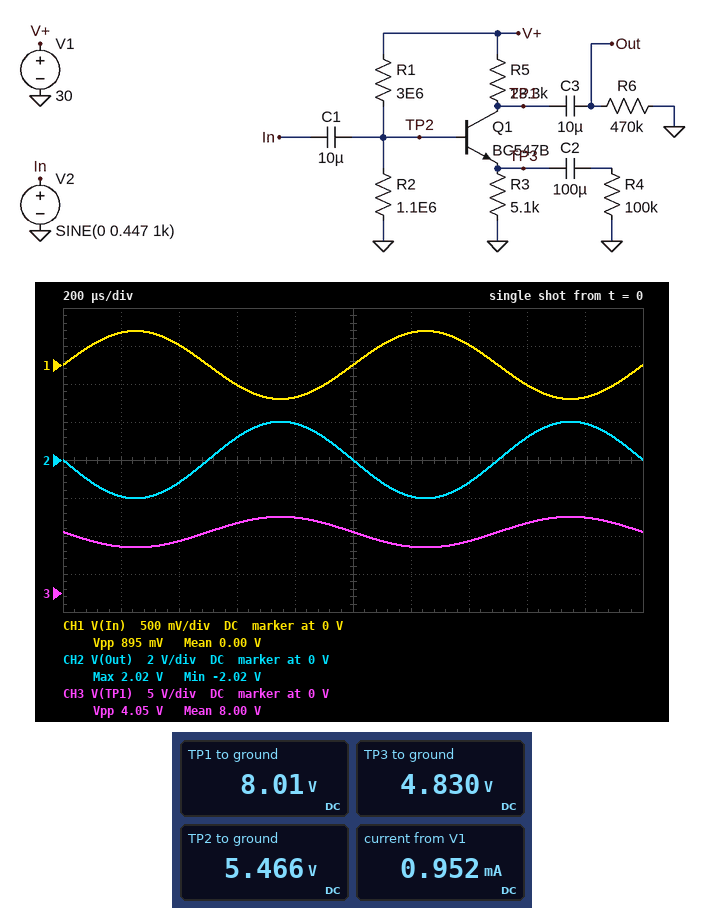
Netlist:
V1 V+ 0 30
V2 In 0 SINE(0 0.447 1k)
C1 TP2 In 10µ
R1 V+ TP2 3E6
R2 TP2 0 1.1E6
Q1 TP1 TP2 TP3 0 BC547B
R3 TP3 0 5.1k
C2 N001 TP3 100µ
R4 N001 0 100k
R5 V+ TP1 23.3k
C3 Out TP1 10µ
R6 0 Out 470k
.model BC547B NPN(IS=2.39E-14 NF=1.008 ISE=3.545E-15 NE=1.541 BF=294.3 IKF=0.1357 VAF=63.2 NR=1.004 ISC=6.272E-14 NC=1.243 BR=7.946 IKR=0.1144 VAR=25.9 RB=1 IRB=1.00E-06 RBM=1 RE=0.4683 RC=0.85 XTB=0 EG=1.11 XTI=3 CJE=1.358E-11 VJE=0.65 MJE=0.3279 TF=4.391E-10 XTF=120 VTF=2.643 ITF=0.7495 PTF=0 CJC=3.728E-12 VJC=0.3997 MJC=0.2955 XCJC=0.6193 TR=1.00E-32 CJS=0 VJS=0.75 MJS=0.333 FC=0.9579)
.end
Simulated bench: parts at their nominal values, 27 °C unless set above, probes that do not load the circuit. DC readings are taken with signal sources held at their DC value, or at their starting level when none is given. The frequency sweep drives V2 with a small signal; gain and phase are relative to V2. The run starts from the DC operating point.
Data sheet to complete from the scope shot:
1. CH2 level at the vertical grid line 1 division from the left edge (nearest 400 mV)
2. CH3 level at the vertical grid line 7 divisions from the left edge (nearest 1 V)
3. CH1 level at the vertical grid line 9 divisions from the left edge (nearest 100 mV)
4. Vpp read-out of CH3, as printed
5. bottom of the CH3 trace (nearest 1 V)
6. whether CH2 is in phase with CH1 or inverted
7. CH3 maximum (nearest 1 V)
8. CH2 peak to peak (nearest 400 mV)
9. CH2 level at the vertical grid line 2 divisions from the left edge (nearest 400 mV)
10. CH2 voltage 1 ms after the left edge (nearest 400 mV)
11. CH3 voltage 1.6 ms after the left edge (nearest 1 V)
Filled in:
-2.0 V
7 V
-400 mV
4.05 V
6 V
inverted
10 V
4.0 V
-1.2 V
0 V
9 V
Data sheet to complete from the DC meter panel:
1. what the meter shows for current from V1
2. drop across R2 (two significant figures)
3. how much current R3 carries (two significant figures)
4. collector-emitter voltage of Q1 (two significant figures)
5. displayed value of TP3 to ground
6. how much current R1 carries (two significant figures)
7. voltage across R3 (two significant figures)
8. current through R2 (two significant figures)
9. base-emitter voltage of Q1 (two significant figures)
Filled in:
0.952 mA
5.5 V
950 µA
3.2 V
4.830 V
8.2 µA
4.8 V
5.0 µA
640 mV
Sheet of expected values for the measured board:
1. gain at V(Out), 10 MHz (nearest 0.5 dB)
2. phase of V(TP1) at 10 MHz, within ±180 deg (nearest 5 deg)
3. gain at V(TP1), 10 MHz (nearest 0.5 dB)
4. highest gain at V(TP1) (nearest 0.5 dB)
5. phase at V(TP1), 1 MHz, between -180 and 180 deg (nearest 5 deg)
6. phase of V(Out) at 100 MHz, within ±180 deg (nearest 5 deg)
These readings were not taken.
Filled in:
5.0 dB
70 deg
5.0 dB
13.0 dB
160 deg
5 deg
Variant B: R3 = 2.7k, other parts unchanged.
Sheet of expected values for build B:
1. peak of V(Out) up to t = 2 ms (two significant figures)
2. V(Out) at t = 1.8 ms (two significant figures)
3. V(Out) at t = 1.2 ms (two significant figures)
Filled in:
3.8 V
3.6 V
280 mV
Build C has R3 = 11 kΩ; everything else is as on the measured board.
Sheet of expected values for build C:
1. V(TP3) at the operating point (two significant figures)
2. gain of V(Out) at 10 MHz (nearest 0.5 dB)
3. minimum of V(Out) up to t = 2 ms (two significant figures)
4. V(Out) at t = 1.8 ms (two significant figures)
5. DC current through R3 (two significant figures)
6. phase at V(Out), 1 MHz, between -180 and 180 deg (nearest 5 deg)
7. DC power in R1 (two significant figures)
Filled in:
6.1 V
3.0 dB
-990 mV
940 mV
550 µA
165 deg
180 µW
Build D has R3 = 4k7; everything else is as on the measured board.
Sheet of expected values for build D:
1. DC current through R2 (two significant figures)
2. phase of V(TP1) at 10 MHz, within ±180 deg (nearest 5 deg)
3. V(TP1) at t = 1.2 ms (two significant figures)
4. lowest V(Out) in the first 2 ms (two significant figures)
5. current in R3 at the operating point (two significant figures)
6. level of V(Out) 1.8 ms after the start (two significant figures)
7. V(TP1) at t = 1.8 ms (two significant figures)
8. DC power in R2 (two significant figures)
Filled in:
4.8 µA
70 deg
5.2 V
-1.8 V
990 µA
2.1 V
9.0 V
26 µW
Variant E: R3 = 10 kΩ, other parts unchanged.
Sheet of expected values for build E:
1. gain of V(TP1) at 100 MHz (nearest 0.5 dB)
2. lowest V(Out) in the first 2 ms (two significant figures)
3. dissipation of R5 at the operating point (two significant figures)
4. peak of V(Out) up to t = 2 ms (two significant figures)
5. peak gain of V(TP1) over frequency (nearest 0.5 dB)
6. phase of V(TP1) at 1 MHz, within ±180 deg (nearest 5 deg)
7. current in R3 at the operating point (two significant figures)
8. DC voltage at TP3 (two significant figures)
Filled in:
0.5 dB
-1.1 V
8.2 mW
1.1 V
7.5 dB
165 deg
600 µA
6.0 V
